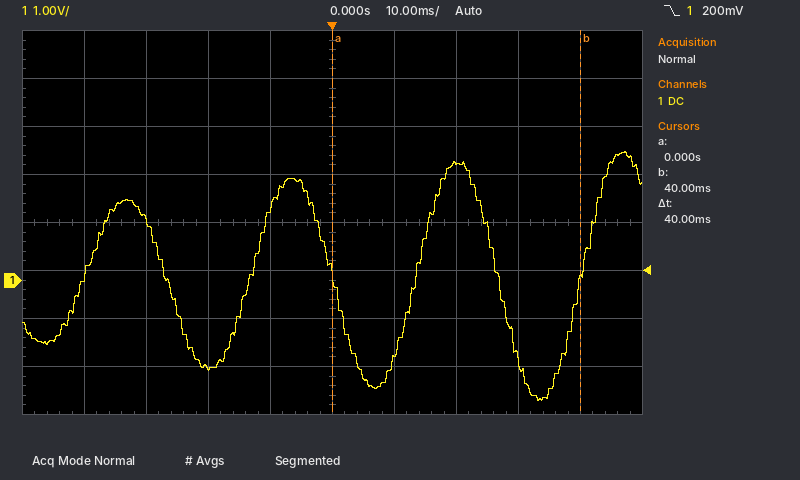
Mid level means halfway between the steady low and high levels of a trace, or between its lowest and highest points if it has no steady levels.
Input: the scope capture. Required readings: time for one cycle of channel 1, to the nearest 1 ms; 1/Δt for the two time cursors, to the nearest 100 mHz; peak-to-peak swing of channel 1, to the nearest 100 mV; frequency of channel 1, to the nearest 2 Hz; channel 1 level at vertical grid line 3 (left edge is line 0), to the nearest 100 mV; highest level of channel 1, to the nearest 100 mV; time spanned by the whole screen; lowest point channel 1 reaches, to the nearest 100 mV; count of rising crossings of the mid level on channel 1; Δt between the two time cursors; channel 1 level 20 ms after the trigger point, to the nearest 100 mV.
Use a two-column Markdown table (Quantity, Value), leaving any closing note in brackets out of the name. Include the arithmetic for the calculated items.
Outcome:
| Quantity | Value |
|---|---|
| time for one cycle of channel 1, to the nearest 1 ms | 27 ms |
| 1/Δt for the two time cursors, to the nearest 100 mHz | 1 / 40 ms ≈ 25.0 Hz |
| peak-to-peak swing of channel 1, to the nearest 100 mV | 2.7 V − (-2.5 V) = 5.2 V |
| frequency of channel 1, to the nearest 2 Hz | 1 / 27 ms ≈ 37.0 Hz, so 38 Hz to the nearest 2 Hz |
| channel 1 level at vertical grid line 3 (left edge is line 0), to the nearest 100 mV | -1.8 V |
| highest level of channel 1, to the nearest 100 mV | 2.7 V |
| time spanned by the whole screen | 100 ms |
| lowest point channel 1 reaches, to the nearest 100 mV | -2.5 V |
| count of rising crossings of the mid level on channel 1 | 4 |
| Δt between the two time cursors | 40 ms |
| channel 1 level 20 ms after the trigger point, to the nearest 100 mV | 2.4 V |
